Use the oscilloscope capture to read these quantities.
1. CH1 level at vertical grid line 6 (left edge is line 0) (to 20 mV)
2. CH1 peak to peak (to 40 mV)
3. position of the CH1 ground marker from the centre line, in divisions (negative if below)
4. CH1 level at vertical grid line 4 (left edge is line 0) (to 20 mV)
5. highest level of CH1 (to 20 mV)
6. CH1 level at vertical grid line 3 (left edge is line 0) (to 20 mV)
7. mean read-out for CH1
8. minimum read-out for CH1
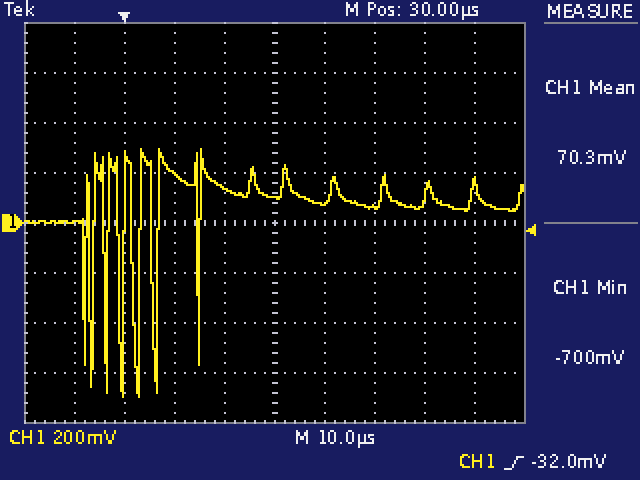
80 mV
1.00 V
0.0 div
140 mV
300 mV
200 mV
70.3 mV
-700 mV
